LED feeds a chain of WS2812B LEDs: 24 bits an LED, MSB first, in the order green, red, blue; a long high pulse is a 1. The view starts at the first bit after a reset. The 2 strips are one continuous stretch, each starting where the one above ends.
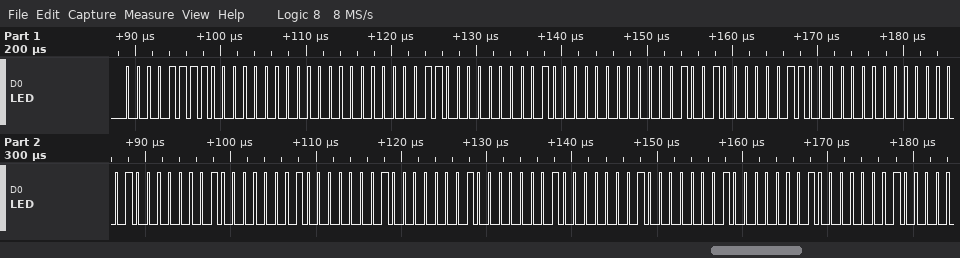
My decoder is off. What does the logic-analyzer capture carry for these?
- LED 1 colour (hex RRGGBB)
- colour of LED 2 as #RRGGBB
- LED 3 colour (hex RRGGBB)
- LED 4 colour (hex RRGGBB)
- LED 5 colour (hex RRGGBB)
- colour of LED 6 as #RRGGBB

#000F00
#010C00
#030900
#010101
#010101
#010101
